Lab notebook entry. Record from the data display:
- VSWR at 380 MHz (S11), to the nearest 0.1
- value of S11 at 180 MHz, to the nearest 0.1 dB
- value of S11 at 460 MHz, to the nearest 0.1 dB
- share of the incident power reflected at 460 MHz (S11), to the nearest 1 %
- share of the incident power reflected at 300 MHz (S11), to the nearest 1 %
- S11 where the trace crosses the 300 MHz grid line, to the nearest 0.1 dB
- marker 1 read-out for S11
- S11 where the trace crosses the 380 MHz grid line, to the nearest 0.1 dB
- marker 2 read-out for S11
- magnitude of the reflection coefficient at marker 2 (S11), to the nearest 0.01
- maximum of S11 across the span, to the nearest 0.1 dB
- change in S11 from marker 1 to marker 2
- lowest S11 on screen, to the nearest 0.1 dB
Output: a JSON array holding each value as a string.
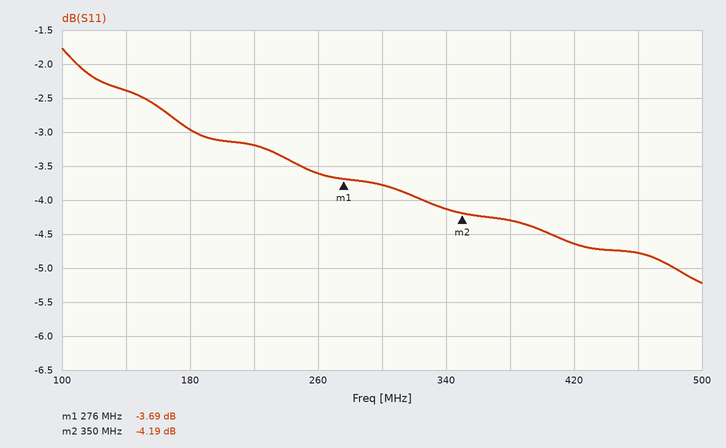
["4.1", "-3.0 dB", "-4.8 dB", "33 %", "42 %", "-3.8 dB", "-3.69 dB", "-4.3 dB", "-4.19 dB", "0.62", "-1.8 dB", "-0.50 dB", "-5.2 dB"]
